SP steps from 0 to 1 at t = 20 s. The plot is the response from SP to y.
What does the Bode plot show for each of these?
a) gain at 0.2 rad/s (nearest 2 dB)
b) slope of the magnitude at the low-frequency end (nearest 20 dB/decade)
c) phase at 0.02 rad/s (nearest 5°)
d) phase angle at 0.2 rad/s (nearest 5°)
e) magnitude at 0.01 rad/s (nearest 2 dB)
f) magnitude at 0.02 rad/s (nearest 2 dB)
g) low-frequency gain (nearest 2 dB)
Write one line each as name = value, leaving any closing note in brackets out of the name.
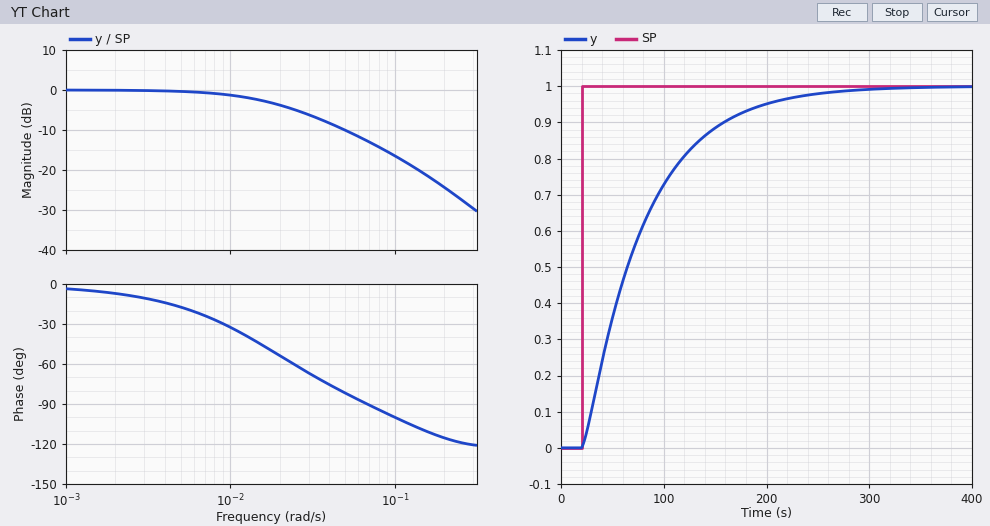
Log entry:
gain at 0.2 rad/s = -24 dB
slope of the magnitude at the low-frequency end = 0 dB/decade
phase at 0.02 rad/s = -55°
phase angle at 0.2 rad/s = -115°
magnitude at 0.01 rad/s = -2 dB
magnitude at 0.02 rad/s = -4 dB
low-frequency gain = 0 dB
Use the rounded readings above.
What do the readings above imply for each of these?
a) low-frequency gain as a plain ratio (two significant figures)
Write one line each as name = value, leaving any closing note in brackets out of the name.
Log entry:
low-frequency gain as a plain ratio = 1.0
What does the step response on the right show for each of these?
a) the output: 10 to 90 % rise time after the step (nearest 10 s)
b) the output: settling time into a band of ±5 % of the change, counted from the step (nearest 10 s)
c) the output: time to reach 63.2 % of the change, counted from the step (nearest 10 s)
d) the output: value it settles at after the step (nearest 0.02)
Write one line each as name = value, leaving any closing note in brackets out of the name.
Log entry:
the output: 10 to 90 % rise time after the step = 130 s
the output: settling time into a band of ±5 % of the change, counted from the step = 180 s
the output: time to reach 63.2 % of the change, counted from the step = 60 s
the output: value it settles at after the step = 1.00
